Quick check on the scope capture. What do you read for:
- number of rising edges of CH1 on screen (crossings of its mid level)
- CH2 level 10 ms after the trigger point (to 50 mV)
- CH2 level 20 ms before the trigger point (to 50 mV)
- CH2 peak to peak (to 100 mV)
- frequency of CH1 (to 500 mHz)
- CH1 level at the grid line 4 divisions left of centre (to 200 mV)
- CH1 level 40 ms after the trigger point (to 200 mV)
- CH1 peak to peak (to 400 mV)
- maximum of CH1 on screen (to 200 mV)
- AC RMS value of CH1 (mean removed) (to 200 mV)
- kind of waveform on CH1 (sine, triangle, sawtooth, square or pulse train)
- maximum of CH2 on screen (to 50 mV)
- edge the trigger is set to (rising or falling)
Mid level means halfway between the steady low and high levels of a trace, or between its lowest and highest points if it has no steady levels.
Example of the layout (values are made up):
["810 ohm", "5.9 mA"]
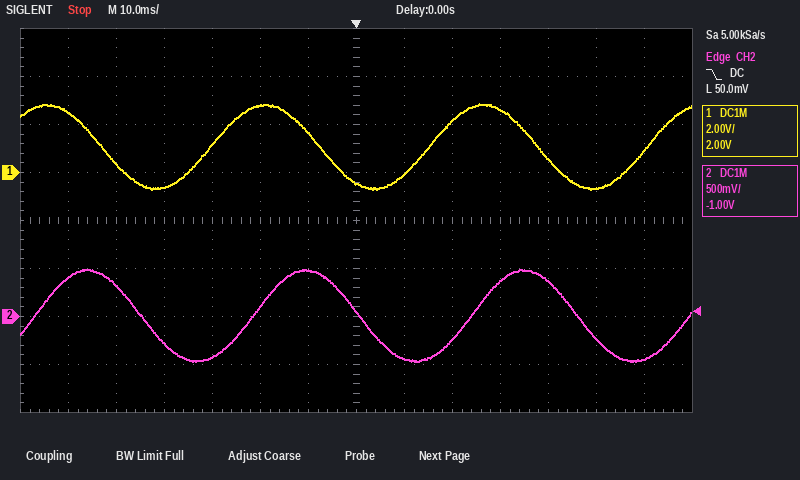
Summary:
["3", "-450 mV", "100 mV", "1.00 V", "22.0 Hz", "-600 mV", "600 mV", "3.6 V", "2.8 V", "1.2 V", "sine", "500 mV", "falling"]
